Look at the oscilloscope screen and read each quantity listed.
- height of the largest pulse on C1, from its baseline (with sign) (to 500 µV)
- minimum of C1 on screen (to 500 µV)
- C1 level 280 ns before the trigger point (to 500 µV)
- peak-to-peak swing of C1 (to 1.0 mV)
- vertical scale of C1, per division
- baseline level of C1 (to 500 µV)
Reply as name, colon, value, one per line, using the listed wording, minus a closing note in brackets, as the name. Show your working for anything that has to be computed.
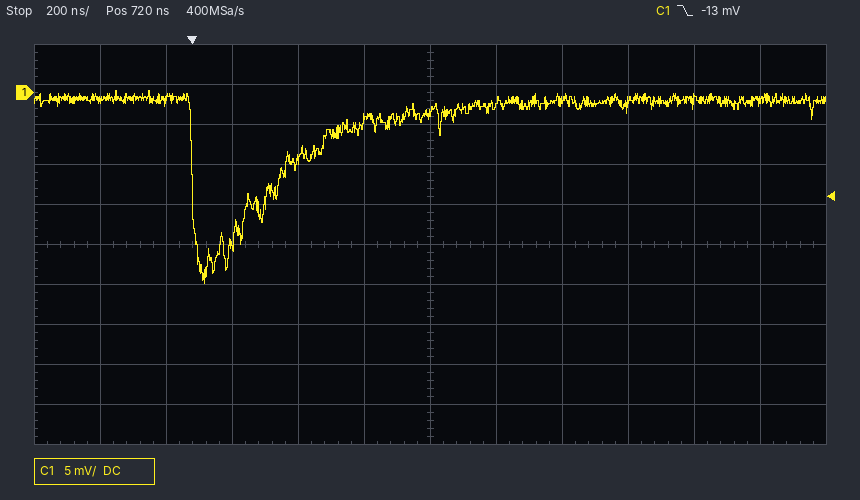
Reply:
height of the largest pulse on C1, from its baseline (with sign): -24.0 mV − (-1.0 mV) = -23.0 mV
minimum of C1 on screen: -24.0 mV
C1 level 280 ns before the trigger point: -1.0 mV
peak-to-peak swing of C1: 24.0 mV
vertical scale of C1, per division: 5 mV
baseline level of C1: -1.0 mV
